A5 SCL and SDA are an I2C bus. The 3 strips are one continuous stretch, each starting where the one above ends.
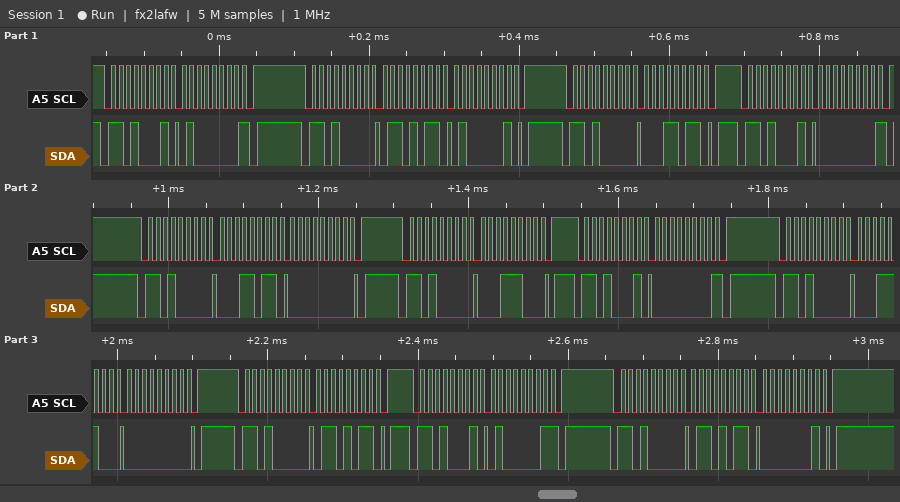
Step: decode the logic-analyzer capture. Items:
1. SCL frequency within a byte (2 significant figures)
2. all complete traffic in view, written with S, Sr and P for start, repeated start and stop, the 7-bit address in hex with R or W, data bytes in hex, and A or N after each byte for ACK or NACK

100 kHz
S 68R A 40 N P S 68W A 6B A 41 A P S 68W A 1B A P S 68R A 00 N P S 68W A 1B A 00 A P S 68W A 1C A P S 68R A 00 N P S 68W A 1C A 00 A P S 68W A 6B A P S 68R A 41 N P S 68W A 6B A 01 A P
